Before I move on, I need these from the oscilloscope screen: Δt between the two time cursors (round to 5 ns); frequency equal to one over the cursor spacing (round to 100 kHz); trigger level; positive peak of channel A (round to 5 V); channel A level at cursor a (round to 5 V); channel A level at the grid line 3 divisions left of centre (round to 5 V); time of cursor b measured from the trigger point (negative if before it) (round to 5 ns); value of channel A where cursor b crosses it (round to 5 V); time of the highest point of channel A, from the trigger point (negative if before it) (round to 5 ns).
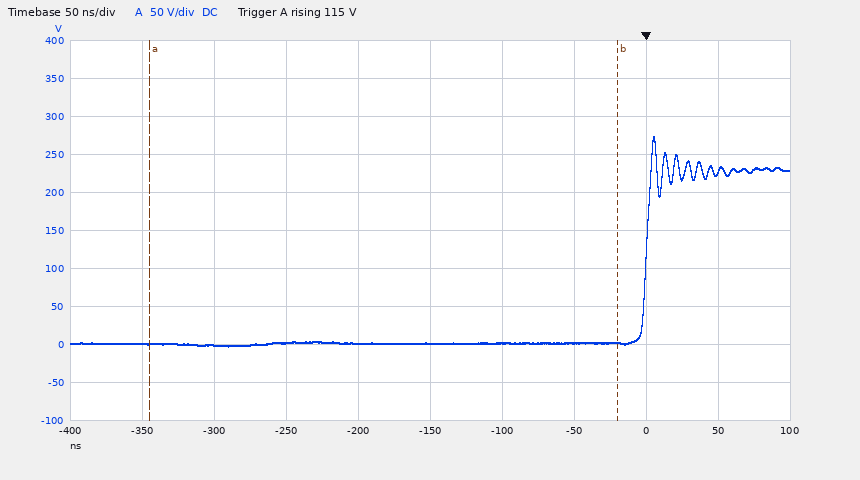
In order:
325 ns
3.1 MHz
115 V
275 V
0 V
0 V
-20 ns
0 V
+5 ns
